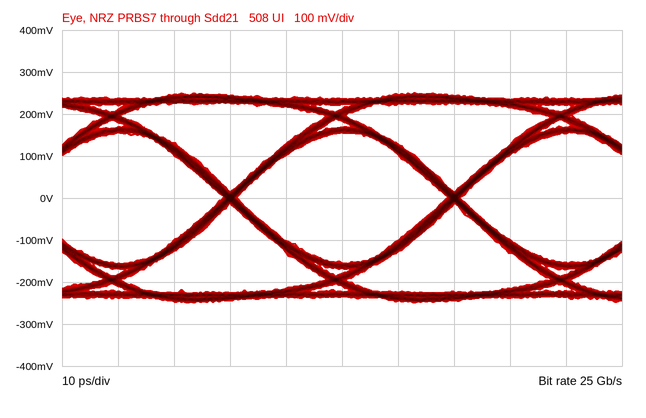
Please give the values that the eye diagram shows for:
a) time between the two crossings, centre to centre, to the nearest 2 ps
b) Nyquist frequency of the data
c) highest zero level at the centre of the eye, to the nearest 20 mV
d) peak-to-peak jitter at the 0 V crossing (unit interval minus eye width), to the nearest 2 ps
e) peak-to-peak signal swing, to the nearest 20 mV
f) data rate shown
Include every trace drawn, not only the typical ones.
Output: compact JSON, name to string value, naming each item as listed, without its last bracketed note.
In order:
{"time between the two crossings, centre to centre, to the nearest 2 ps": "40 ps", "Nyquist frequency of the data": "12.5 GHz", "highest zero level at the centre of the eye, to the nearest 20 mV": "-160 mV", "peak-to-peak jitter at the 0 V crossing (unit interval minus eye width), to the nearest 2 ps": "2 ps", "peak-to-peak signal swing, to the nearest 20 mV": "500 mV", "data rate shown": "25 Gb/s"}
